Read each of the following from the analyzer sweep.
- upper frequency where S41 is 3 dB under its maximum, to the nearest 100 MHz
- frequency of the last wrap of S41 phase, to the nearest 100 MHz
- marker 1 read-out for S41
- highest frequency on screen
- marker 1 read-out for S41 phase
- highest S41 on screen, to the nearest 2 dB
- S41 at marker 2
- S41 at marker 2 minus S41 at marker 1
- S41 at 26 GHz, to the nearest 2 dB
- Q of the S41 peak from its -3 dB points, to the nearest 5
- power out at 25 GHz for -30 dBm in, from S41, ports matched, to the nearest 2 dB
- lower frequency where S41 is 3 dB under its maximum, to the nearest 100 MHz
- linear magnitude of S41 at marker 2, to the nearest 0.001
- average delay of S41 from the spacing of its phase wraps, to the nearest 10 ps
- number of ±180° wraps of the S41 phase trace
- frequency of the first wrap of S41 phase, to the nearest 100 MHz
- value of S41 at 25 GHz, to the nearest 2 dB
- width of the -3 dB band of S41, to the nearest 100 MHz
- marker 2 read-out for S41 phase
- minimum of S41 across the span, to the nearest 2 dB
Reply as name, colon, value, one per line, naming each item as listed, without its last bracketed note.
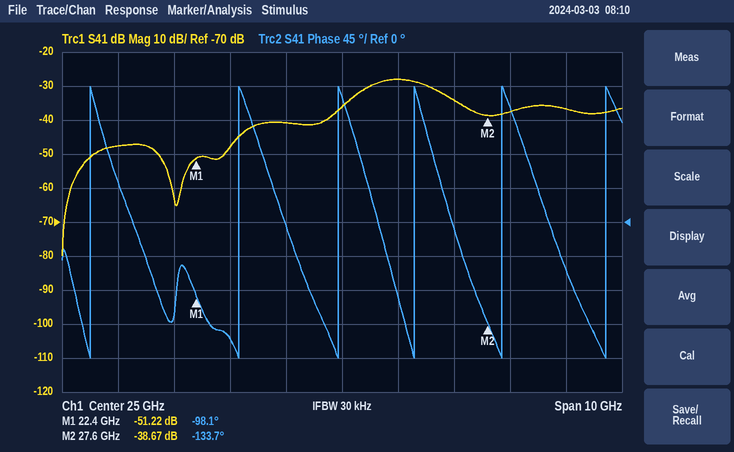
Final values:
upper frequency where S41 is 3 dB under its maximum, to the nearest 100 MHz: 26.7 GHz
frequency of the last wrap of S41 phase, to the nearest 100 MHz: 29.7 GHz
marker 1 read-out for S41: -51.22 dB
highest frequency on screen: 30 GHz
marker 1 read-out for S41 phase: -98.1°
highest S41 on screen, to the nearest 2 dB: -28 dB
S41 at marker 2: -38.67 dB
S41 at marker 2 minus S41 at marker 1: 12.55 dB
S41 at 26 GHz, to the nearest 2 dB: -28 dB
Q of the S41 peak from its -3 dB points, to the nearest 5: 20
power out at 25 GHz for -30 dBm in, from S41, ports matched, to the nearest 2 dB: -66 dBm
lower frequency where S41 is 3 dB under its maximum, to the nearest 100 MHz: 25.4 GHz
linear magnitude of S41 at marker 2, to the nearest 0.001: 0.012
average delay of S41 from the spacing of its phase wraps, to the nearest 10 ps: 540 ps
number of ±180° wraps of the S41 phase trace: 6
frequency of the first wrap of S41 phase, to the nearest 100 MHz: 20.5 GHz
value of S41 at 25 GHz, to the nearest 2 dB: -36 dB
width of the -3 dB band of S41, to the nearest 100 MHz: 1.3 GHz
marker 2 read-out for S41 phase: -133.7°
minimum of S41 across the span, to the nearest 2 dB: -80 dB
